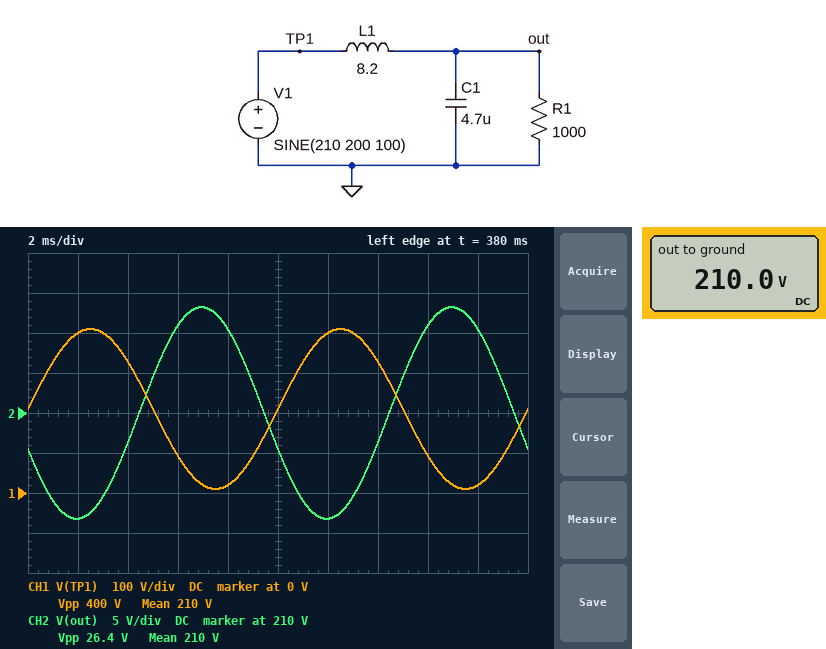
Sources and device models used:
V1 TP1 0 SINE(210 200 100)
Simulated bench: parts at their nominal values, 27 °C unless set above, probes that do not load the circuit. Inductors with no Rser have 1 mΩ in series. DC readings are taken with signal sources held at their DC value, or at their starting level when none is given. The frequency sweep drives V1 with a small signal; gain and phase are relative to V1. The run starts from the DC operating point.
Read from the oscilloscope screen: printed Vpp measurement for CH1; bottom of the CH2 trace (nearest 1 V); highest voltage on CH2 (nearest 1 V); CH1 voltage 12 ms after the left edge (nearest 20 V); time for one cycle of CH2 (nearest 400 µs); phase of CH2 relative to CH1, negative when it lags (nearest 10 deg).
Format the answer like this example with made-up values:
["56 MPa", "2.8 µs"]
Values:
["400 V", "197 V", "223 V", "400 V", "10.0 ms", "-160 deg"]
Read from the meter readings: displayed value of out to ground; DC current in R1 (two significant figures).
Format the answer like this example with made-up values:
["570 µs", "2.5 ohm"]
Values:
["210.0 V", "210 mA"]
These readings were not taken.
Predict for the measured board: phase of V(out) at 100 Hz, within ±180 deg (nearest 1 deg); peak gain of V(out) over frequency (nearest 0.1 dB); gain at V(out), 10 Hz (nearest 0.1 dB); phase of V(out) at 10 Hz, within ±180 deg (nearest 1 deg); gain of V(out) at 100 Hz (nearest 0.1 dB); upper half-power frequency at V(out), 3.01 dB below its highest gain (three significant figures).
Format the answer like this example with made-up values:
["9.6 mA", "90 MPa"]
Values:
["-160 deg", "0.1 dB", "0.1 dB", "-31 deg", "-23.6 dB", "27.1 Hz"]
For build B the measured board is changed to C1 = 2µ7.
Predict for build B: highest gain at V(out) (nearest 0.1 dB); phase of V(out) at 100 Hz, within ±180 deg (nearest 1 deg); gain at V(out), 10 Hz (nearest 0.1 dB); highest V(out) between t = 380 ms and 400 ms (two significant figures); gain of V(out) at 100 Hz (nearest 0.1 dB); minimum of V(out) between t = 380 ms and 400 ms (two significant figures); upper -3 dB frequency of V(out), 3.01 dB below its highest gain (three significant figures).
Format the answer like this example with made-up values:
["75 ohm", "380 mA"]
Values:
["0 dB", "-146 deg", "-0.4 dB", "230 V", "-19.4 dB", "190 V", "26.4 Hz"]
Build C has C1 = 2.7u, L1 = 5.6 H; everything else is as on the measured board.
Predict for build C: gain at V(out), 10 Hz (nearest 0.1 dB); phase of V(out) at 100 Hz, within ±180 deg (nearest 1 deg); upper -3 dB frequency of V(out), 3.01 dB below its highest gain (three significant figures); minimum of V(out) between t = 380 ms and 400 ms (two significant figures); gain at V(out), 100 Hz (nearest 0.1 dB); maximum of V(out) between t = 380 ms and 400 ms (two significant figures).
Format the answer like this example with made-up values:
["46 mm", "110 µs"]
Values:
["0 dB", "-145 deg", "40.2 Hz", "180 V", "-15.7 dB", "240 V"]
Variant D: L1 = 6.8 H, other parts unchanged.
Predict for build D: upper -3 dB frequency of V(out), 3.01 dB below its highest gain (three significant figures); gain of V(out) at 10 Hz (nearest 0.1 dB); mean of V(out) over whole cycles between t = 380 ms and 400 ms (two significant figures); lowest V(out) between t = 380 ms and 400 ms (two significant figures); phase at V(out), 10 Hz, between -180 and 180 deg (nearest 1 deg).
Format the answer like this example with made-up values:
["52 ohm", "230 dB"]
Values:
["31.3 Hz", "0.2 dB", "210 V", "190 V", "-26 deg"]
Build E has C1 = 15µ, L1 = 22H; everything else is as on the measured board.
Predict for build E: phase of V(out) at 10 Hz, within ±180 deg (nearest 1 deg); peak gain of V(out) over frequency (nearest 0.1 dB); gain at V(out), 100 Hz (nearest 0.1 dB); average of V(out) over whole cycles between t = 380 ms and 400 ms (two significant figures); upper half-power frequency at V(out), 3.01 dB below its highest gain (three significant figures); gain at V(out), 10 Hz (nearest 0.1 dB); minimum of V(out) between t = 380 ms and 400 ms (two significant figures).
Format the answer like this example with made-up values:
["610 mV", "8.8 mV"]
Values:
["-102 deg", "0.3 dB", "-42.3 dB", "210 V", "9.72 Hz", "-3.0 dB", "210 V"]
